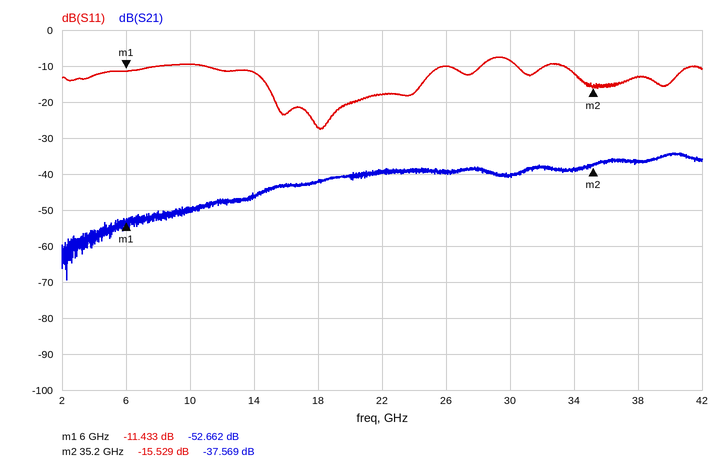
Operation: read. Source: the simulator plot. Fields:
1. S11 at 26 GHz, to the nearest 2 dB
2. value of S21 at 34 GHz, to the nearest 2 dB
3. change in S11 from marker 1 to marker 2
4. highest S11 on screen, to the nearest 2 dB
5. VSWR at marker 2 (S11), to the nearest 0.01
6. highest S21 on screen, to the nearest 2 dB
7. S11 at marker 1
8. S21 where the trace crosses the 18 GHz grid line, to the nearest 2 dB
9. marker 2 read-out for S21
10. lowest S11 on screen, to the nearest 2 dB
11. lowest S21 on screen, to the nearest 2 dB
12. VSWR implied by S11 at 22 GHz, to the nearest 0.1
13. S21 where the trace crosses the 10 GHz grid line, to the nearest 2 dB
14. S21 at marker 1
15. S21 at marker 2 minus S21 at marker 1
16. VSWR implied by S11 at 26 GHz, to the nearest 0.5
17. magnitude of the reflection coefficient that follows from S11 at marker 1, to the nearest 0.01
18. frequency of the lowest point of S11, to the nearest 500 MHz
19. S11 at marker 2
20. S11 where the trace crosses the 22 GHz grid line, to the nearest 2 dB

-10 dB
-38 dB
-4.096 dB
-8 dB
1.40
-34 dB
-11.433 dB
-42 dB
-37.569 dB
-28 dB
-70 dB
1.3
-50 dB
-52.662 dB
15.093 dB
2.0
0.27
18.0 GHz
-15.529 dB
-18 dB
